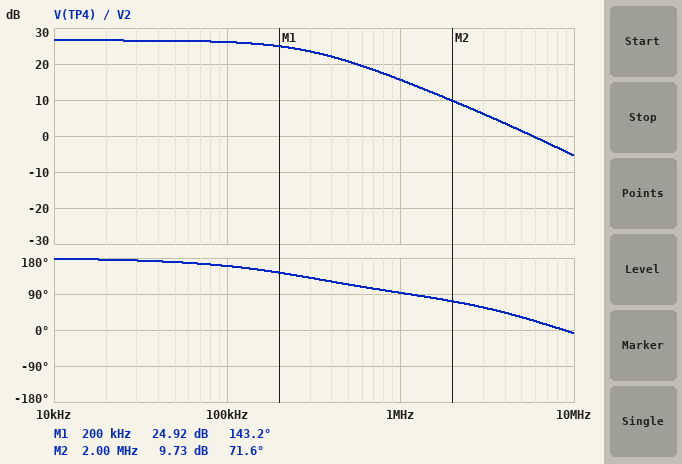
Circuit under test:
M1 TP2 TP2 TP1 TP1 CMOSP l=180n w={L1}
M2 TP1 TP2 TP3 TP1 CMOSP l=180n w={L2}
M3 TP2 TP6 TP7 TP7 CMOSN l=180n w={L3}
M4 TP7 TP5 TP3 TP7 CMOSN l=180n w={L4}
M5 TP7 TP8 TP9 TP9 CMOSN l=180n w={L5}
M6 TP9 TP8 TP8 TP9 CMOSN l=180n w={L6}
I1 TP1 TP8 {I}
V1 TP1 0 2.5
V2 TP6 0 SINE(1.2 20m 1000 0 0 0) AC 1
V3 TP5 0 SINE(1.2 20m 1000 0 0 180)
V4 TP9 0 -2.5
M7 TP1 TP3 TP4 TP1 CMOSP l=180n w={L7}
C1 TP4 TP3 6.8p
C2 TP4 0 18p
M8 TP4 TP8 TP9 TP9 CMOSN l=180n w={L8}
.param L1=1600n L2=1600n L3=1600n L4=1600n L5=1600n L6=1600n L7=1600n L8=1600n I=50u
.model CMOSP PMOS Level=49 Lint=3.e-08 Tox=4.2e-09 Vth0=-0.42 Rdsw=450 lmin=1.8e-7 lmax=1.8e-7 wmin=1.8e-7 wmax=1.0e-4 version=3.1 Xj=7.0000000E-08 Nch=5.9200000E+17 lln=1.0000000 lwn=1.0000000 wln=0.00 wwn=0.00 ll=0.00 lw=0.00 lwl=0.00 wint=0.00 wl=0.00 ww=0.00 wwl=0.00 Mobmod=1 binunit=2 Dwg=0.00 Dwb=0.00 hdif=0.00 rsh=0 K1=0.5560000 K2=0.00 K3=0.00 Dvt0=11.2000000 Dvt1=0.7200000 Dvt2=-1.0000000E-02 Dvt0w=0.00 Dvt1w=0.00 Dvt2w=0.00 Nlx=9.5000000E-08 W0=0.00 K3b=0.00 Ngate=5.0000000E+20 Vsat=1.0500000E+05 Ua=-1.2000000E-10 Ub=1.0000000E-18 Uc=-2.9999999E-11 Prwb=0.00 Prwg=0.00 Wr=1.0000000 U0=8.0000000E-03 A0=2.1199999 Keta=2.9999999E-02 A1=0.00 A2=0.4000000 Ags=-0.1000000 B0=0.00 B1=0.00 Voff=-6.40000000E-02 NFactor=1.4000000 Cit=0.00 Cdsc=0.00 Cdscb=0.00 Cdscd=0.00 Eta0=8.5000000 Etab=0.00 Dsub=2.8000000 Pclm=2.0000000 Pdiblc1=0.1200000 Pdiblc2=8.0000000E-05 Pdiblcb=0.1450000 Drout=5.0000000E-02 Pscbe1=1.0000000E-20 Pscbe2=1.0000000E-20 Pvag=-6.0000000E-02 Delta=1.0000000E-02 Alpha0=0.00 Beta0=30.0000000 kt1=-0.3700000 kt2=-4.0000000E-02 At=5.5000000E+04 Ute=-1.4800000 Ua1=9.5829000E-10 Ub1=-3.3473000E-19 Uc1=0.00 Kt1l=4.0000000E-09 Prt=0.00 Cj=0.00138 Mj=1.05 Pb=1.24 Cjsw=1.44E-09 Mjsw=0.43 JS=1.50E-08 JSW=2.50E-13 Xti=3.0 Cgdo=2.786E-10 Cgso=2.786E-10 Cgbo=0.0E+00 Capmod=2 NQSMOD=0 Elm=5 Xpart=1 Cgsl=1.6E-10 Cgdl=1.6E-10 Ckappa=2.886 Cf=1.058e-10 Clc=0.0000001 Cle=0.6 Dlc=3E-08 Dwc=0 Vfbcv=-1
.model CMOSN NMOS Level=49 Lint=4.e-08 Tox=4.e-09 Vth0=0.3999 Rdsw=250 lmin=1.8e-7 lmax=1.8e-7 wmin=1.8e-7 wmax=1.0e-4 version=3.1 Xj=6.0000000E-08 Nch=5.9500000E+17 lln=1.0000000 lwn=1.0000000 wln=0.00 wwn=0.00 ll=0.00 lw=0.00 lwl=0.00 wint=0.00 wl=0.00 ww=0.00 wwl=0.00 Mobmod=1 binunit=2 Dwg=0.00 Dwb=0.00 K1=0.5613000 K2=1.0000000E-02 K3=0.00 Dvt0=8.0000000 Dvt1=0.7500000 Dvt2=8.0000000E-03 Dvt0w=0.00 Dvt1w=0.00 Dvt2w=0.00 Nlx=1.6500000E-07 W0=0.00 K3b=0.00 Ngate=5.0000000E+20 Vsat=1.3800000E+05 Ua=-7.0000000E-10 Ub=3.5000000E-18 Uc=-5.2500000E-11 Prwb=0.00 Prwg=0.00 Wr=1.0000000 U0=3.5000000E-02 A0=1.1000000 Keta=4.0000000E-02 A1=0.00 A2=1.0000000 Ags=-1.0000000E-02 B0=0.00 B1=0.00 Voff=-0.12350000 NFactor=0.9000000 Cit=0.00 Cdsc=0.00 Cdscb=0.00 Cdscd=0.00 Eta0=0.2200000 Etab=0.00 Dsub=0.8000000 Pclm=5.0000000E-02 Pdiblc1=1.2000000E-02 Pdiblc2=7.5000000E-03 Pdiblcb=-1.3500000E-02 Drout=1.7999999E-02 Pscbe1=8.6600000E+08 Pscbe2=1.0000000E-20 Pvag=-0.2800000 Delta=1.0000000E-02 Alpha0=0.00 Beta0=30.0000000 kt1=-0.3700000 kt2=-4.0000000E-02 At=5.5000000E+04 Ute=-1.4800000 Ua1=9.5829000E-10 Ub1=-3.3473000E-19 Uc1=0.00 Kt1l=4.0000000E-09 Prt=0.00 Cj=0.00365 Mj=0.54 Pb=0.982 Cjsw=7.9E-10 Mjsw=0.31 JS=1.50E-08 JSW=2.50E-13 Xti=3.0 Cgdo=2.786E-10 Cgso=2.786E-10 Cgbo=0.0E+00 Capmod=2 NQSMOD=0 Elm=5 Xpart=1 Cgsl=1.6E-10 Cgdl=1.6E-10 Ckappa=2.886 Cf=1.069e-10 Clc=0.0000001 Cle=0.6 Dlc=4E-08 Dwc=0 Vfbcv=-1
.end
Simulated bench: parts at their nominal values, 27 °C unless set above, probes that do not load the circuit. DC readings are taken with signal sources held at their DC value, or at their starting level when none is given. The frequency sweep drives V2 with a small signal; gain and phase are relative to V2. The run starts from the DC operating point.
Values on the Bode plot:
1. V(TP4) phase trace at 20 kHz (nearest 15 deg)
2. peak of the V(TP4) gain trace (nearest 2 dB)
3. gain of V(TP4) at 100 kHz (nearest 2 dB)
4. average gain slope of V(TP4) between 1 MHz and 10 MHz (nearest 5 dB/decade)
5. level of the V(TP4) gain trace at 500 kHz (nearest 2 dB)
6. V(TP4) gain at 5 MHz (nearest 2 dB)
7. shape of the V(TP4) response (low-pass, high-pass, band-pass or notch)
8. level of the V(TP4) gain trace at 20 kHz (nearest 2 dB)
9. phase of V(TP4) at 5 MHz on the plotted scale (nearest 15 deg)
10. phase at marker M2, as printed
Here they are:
180 deg
26 dB
26 dB
-20 dB/decade
20 dB
2 dB
low-pass
26 dB
30 deg
71.6 deg
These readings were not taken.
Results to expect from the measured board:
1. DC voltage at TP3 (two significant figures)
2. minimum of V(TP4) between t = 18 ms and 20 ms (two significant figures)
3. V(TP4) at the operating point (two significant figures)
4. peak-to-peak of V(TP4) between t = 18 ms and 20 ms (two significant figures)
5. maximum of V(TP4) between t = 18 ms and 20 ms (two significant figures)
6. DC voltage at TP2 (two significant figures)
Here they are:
1.7 V
-870 mV
150 mV
1.8 V
900 mV
1.7 V
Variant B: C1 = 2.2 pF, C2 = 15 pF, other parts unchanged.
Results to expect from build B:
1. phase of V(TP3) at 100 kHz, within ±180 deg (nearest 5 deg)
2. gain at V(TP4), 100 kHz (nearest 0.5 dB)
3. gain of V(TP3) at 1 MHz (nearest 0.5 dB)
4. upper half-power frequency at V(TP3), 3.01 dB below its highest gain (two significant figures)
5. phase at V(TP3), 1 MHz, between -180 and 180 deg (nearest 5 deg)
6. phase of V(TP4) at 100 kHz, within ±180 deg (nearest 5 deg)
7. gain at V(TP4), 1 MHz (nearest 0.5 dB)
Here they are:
-5 deg
26.5 dB
12.5 dB
1.2 MHz
-20 deg
170 deg
21.0 dB
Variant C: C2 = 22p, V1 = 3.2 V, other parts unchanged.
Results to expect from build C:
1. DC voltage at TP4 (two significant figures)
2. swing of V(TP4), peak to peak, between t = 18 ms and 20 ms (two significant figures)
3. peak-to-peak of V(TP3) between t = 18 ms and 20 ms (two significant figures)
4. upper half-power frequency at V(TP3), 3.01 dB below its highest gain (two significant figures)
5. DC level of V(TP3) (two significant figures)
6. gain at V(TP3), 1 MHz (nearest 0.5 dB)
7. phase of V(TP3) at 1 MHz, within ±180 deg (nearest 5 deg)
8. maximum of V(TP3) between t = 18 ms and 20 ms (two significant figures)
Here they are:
430 mV
1.9 V
480 mV
350 kHz
2.4 V
9.5 dB
-25 deg
2.6 V
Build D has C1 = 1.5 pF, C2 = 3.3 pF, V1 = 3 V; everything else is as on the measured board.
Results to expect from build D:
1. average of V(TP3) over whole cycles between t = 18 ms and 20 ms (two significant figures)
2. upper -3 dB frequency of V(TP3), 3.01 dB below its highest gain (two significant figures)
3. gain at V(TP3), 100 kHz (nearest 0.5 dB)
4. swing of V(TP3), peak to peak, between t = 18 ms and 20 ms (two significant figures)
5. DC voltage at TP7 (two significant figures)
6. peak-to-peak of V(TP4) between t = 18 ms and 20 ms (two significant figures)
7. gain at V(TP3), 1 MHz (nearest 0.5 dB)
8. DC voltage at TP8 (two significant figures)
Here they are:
2.2 V
1.6 MHz
15.5 dB
480 mV
640 mV
1.9 V
14.0 dB
-1.9 V
